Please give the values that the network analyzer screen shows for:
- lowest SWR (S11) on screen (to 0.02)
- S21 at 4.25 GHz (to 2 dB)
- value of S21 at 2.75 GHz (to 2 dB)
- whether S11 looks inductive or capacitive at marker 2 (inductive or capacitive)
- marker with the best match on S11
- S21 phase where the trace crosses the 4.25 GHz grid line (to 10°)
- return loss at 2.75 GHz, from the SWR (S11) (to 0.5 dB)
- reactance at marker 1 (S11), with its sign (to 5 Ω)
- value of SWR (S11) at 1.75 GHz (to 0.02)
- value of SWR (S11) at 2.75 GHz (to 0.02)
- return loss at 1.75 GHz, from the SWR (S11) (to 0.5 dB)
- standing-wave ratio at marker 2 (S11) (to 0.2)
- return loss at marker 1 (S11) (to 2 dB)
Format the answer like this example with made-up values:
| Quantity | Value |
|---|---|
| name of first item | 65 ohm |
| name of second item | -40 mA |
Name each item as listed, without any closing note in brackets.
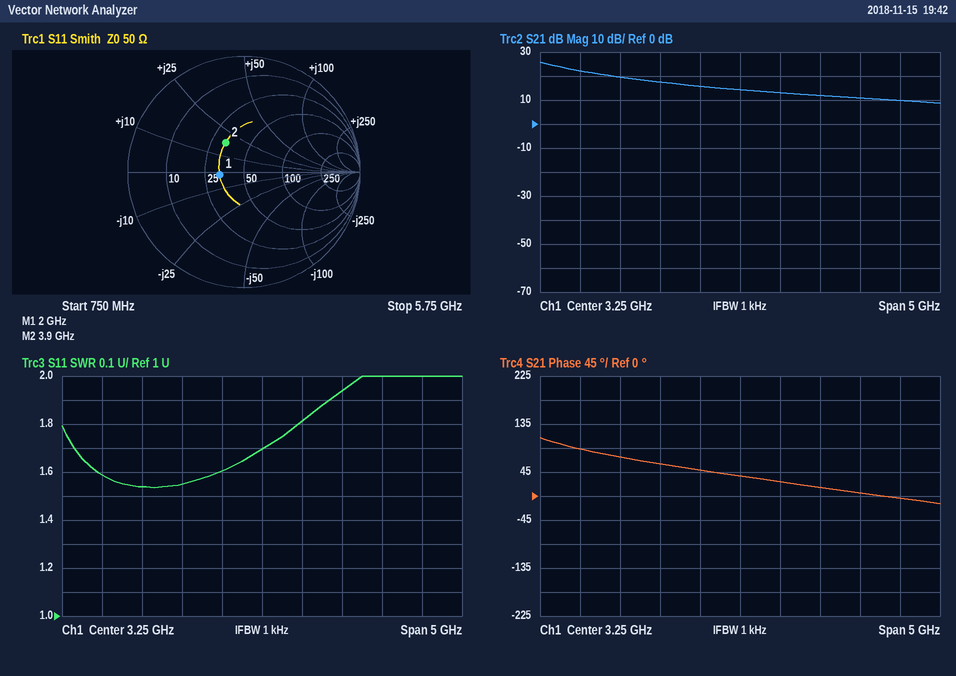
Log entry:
| Quantity | Value |
|---|---|
| lowest SWR (S11) on screen | 1.54 |
| S21 at 4.25 GHz | 12 dB |
| value of S21 at 2.75 GHz | 16 dB |
| whether S11 looks inductive or capacitive at marker 2 | inductive |
| marker with the best match on S11 | marker 1 |
| S21 phase where the trace crosses the 4.25 GHz grid line | 20° |
| return loss at 2.75 GHz, from the SWR (S11) | 12.5 dB |
| reactance at marker 1 (S11), with its sign | 0 Ω |
| value of SWR (S11) at 1.75 GHz | 1.54 |
| value of SWR (S11) at 2.75 GHz | 1.60 |
| return loss at 1.75 GHz, from the SWR (S11) | 13.5 dB |
| standing-wave ratio at marker 2 (S11) | 1.8 |
| return loss at marker 1 (S11) | 14 dB |
